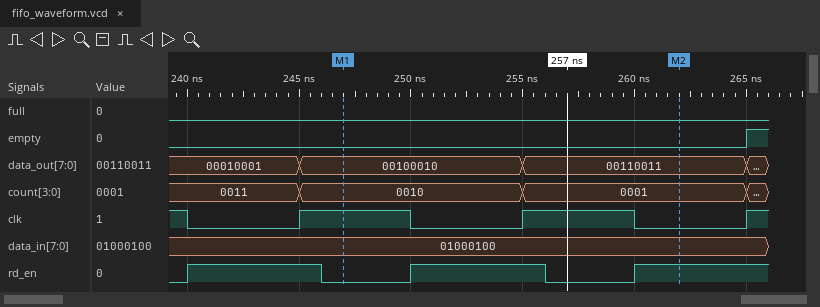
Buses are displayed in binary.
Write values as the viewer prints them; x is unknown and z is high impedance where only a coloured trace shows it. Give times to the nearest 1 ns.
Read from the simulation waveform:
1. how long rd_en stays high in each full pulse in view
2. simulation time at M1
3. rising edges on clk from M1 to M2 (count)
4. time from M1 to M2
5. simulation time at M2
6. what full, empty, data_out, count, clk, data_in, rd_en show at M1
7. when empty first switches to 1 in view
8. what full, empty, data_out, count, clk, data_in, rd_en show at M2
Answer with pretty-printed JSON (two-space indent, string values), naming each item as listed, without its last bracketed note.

{
  "how long rd_en stays high in each full pulse in view": "6 ns, 6 ns",
  "simulation time at M1": "247 ns",
  "rising edges on clk from M1 to M2": "1",
  "time from M1 to M2": "15 ns",
  "simulation time at M2": "262 ns",
  "what full, empty, data_out, count, clk, data_in, rd_en show at M1": "full=0, empty=0, data_out=00100010, count=0010, clk=1, data_in=01000100, rd_en=0",
  "when empty first switches to 1 in view": "265 ns",
  "what full, empty, data_out, count, clk, data_in, rd_en show at M2": "full=0, empty=0, data_out=00110011, count=0001, clk=0, data_in=01000100, rd_en=1"
}
